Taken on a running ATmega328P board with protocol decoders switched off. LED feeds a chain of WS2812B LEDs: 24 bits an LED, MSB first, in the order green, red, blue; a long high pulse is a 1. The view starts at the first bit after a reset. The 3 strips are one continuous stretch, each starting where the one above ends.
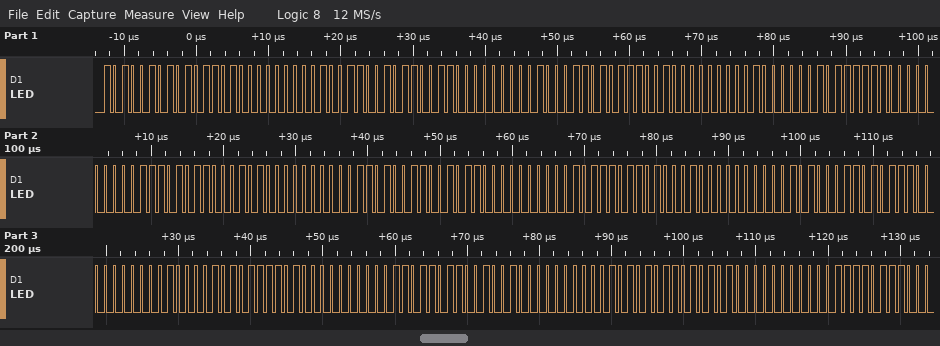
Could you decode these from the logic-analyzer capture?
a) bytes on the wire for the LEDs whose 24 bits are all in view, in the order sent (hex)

A5 5A 00 99 66 00 8D 72 00 81 7E 00 75 8A 00 69 96 00 5D A2 00 51 AE 00 42 BD 00 36 C9 00 2A D5 00
